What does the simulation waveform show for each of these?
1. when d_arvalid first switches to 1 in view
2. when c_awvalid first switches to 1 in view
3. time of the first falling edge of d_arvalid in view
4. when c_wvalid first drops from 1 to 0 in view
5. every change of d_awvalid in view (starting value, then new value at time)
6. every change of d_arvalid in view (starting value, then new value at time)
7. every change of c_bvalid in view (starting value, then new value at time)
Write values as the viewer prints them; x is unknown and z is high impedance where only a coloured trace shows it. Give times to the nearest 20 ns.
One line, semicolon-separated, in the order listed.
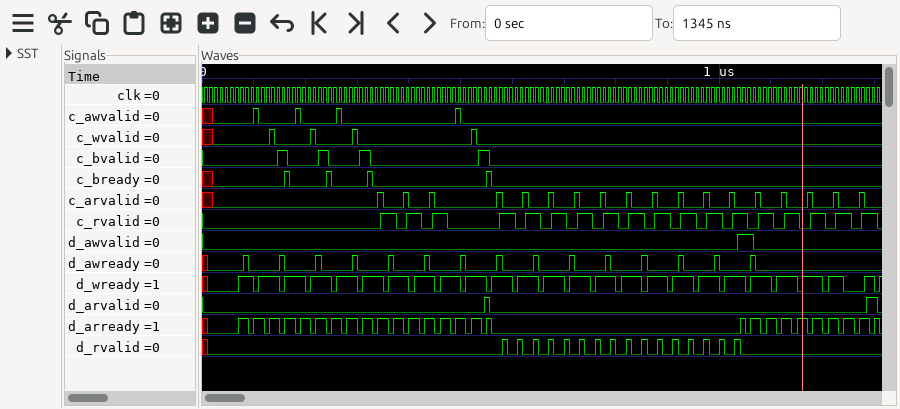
540 ns; 100 ns; 560 ns; 140 ns; 0, 1 at 1040 ns, 0 at 1060 ns; 0, 1 at 540 ns, 0 at 560 ns, 1 at 1280 ns, 0 at 1300 ns; 0, 1 at 140 ns, 0 at 160 ns, 1 at 220 ns, 0 at 240 ns, 1 at 300 ns, 0 at 320 ns, 1 at 540 ns, 0 at 560 ns
